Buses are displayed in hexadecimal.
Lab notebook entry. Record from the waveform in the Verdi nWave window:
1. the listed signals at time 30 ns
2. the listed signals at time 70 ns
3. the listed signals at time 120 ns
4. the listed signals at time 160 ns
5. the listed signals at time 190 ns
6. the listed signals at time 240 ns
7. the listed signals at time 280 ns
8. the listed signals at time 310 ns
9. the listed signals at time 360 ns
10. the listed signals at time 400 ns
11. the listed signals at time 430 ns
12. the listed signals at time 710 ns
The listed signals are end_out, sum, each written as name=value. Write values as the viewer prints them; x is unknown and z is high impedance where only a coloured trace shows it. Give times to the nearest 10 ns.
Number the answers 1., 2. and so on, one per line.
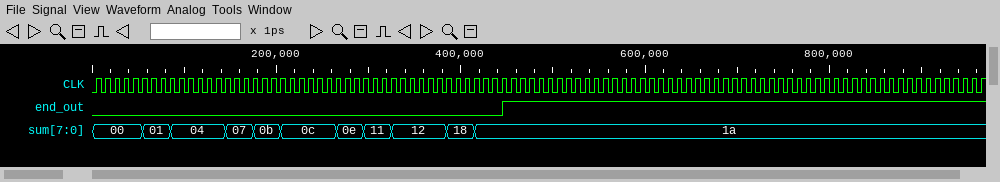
1. end_out=0, sum=00
2. end_out=0, sum=01
3. end_out=0, sum=04
4. end_out=0, sum=07
5. end_out=0, sum=0b
6. end_out=0, sum=0c
7. end_out=0, sum=0e
8. end_out=0, sum=11
9. end_out=0, sum=12
10. end_out=0, sum=18
11. end_out=0, sum=1a
12. end_out=1, sum=1a
